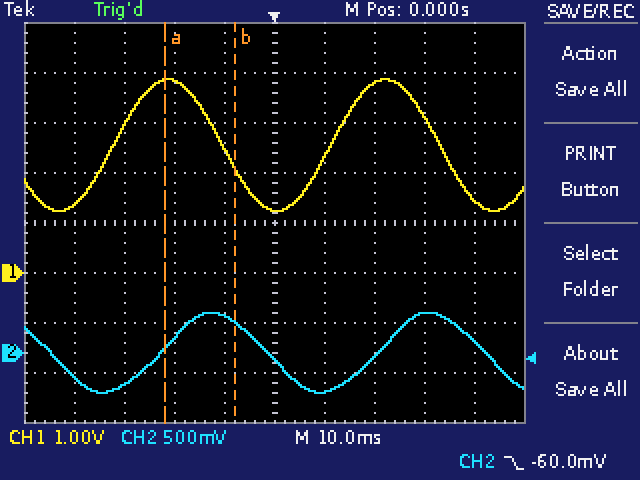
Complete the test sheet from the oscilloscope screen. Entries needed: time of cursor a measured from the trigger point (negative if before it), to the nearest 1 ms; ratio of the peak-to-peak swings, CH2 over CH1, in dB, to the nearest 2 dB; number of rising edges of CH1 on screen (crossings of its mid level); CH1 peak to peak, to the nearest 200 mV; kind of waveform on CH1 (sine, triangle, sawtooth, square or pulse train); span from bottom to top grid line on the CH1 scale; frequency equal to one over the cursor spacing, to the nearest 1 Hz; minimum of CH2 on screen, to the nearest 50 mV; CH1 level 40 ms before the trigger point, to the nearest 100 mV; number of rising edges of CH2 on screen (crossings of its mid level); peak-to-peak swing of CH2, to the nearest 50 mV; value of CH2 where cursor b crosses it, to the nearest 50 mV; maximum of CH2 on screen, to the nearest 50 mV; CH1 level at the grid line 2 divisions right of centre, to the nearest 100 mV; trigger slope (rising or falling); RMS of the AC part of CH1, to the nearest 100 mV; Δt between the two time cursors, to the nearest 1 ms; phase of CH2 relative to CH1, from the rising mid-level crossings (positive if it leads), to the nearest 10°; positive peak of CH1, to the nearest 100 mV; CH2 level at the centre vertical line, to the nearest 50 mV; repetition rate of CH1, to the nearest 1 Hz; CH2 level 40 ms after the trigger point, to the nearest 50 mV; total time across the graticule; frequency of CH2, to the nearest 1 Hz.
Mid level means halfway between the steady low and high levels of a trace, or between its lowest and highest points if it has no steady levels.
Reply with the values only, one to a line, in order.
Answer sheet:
-22 ms
-10 dB
2
2.6 V
sine
8 V
71 Hz
-400 mV
1.4 V
2
800 mV
300 mV
400 mV
3.8 V
falling
900 mV
14 ms
-80°
3.9 V
-50 mV
23 Hz
100 mV
100 ms
23 Hz
